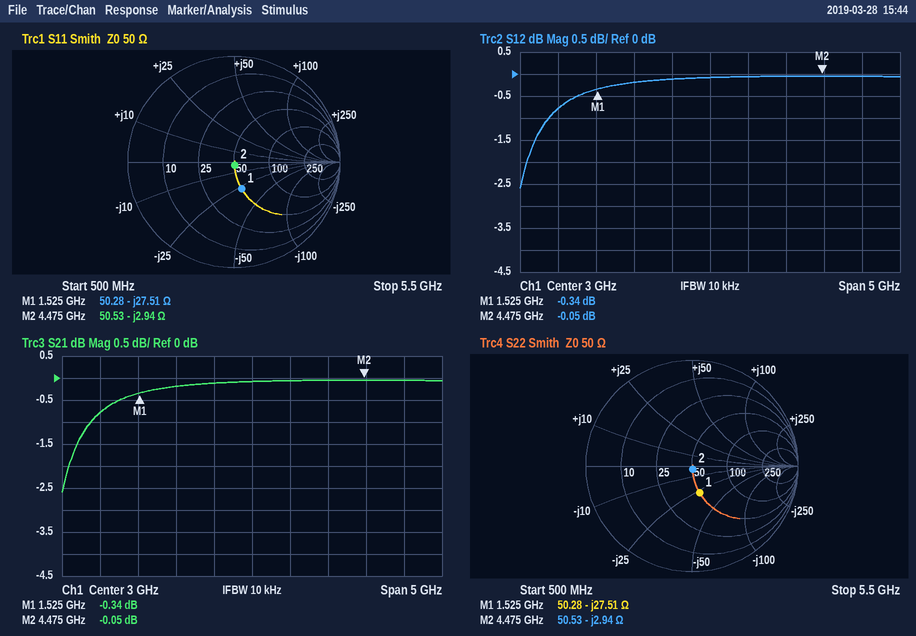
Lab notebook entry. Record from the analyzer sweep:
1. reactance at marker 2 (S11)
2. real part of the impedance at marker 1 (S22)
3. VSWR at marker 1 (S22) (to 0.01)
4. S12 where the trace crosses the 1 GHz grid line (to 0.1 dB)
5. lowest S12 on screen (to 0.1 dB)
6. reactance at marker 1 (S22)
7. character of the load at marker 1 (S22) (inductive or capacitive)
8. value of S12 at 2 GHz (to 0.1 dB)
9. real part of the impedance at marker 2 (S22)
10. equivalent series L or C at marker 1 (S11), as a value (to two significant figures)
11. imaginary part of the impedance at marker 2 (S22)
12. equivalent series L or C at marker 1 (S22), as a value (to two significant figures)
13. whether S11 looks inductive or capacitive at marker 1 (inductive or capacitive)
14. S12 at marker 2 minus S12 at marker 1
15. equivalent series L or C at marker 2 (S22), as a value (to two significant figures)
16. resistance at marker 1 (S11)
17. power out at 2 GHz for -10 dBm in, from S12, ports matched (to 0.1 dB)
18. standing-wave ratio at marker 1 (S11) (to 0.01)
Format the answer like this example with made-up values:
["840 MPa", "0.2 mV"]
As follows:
["-2.94 Ω", "50.28 Ω", "1.72", "-0.8 dB", "-2.6 dB", "-27.51 Ω", "capacitive", "-0.2 dB", "50.53 Ω", "3.8 pF", "-2.94 Ω", "3.8 pF", "capacitive", "0.29 dB", "12 pF", "50.28 Ω", "-10.2 dBm", "1.72"]
